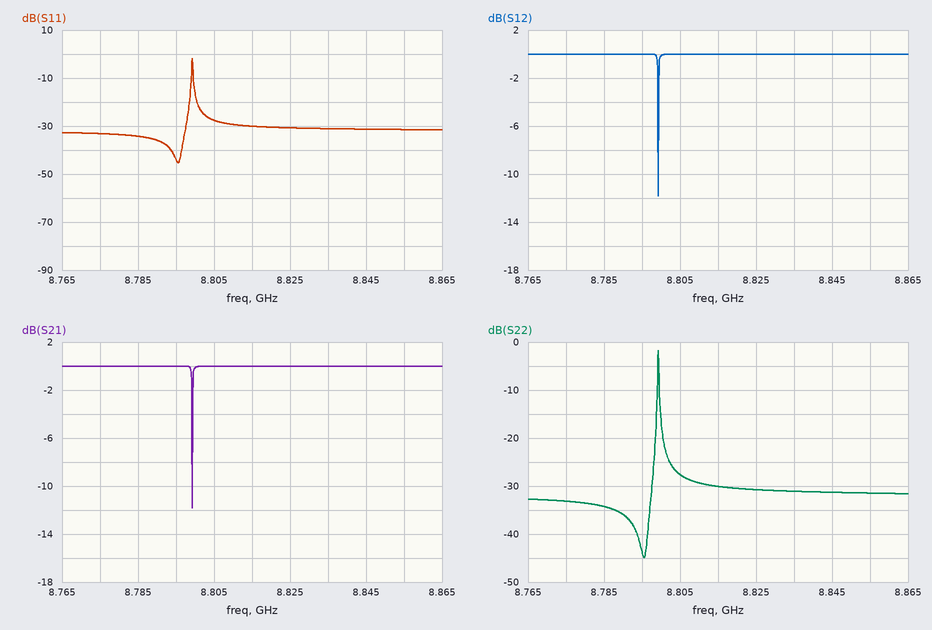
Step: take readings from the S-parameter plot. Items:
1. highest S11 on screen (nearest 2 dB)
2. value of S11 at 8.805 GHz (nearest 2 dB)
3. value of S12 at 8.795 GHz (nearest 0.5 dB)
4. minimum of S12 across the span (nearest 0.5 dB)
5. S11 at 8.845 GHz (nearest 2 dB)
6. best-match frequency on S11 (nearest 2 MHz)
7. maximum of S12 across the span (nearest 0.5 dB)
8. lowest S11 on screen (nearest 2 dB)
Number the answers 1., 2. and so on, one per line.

1. -2 dB
2. -28 dB
3. 0.0 dB
4. -12.0 dB
5. -32 dB
6. 8.796 GHz
7. 0.0 dB
8. -46 dB
